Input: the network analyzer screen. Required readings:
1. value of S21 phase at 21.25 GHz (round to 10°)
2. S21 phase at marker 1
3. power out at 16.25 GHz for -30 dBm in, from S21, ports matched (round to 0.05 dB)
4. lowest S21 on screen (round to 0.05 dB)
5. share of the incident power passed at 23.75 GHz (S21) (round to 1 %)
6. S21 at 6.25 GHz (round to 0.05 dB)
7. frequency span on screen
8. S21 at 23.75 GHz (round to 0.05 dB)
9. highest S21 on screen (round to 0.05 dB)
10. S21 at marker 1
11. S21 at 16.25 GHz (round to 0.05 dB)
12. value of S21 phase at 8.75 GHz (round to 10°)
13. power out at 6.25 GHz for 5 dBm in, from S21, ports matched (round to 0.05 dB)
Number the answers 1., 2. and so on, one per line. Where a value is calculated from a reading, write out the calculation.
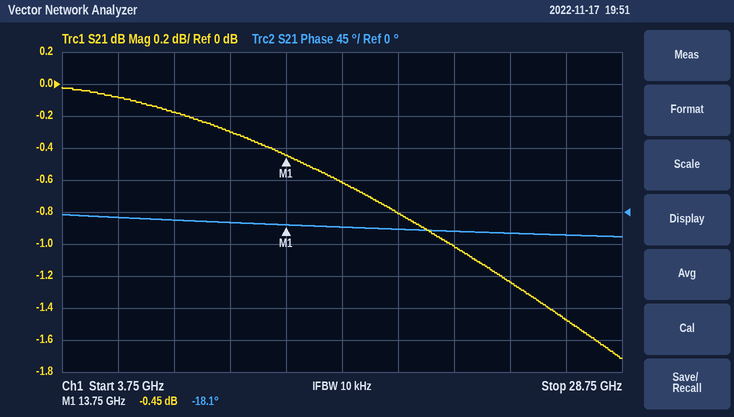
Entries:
1. -30°
2. -18.1°
3. -30 dBm + (-0.60 dB) = -30.60 dBm
4. -1.70 dB
5. 10^(-1.25/10) ≈ 75 %
6. -0.10 dB
7. 25 GHz
8. -1.25 dB
9. 0.00 dB
10. -0.45 dB
11. -0.60 dB
12. -10°
13. 5 dBm + (-0.10 dB) = 4.90 dBm
